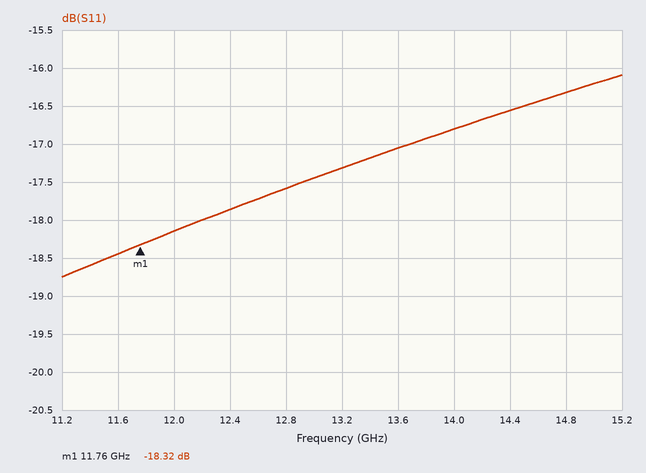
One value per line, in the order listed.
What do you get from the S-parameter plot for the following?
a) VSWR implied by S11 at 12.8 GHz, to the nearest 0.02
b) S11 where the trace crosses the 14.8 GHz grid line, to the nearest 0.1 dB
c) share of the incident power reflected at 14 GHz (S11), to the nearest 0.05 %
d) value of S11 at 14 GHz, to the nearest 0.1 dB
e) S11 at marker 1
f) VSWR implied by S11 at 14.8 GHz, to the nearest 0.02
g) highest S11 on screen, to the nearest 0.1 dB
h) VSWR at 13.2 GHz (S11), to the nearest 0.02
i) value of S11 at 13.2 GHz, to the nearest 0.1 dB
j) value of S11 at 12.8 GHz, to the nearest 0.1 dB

1.30
-16.3 dB
2.10 %
-16.8 dB
-18.32 dB
1.36
-16.1 dB
1.32
-17.3 dB
-17.6 dB
